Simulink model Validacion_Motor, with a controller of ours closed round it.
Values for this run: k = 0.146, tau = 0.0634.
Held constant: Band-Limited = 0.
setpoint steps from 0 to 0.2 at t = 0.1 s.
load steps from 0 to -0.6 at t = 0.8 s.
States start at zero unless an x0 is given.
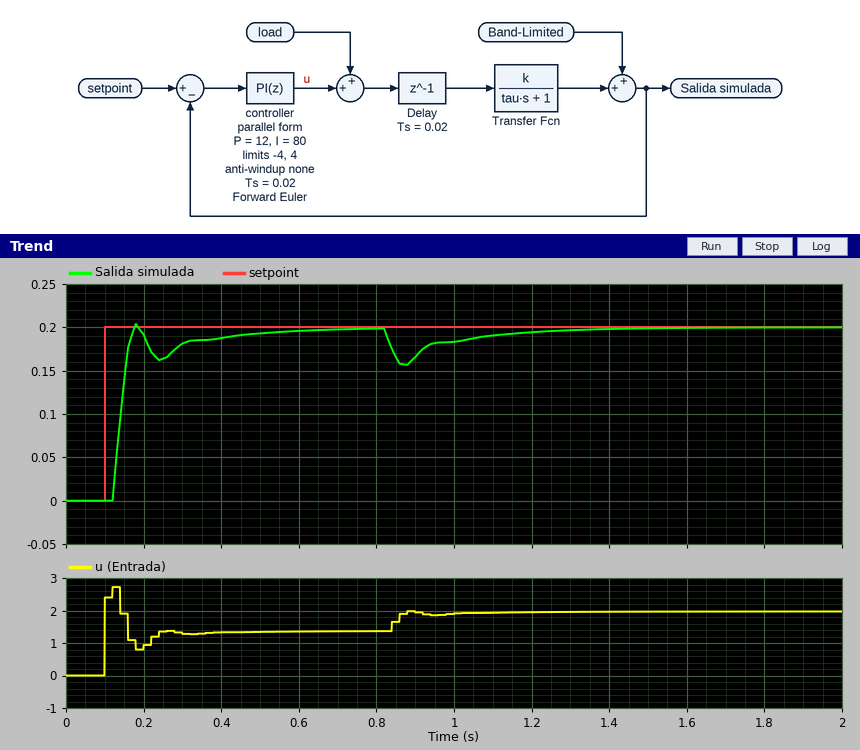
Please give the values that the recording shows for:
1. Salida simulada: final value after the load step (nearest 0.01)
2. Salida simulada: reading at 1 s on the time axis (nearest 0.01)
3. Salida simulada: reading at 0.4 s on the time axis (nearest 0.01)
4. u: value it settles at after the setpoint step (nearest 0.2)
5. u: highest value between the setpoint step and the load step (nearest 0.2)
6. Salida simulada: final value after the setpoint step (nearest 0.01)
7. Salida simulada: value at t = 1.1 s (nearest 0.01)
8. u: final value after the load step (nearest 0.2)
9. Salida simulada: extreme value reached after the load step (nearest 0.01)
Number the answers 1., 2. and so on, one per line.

1. 0.20
2. 0.18
3. 0.19
4. 1.4
5. 2.8
6. 0.20
7. 0.19
8. 2.0
9. 0.16
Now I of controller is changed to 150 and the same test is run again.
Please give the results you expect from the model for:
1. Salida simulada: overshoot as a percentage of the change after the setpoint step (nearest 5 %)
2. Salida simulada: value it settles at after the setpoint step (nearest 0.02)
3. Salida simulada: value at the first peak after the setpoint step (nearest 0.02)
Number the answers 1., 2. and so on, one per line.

1. 20 %
2. 0.20
3. 0.24
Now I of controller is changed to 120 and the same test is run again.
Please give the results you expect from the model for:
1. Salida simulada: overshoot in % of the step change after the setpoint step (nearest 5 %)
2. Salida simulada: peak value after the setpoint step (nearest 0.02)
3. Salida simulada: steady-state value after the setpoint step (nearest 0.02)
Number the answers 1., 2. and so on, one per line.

1. 10 %
2. 0.22
3. 0.20
